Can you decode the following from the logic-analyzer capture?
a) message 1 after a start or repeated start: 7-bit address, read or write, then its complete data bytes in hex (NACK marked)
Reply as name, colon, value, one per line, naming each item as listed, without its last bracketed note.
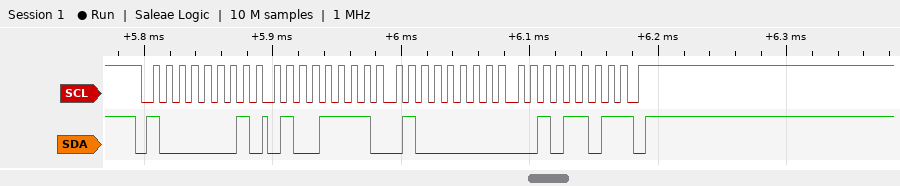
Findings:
message 1 after a start or repeated start: 7-bit address, read or write, then its complete data bytes in hex: 0x40 read: 4F 40 2D NACK
